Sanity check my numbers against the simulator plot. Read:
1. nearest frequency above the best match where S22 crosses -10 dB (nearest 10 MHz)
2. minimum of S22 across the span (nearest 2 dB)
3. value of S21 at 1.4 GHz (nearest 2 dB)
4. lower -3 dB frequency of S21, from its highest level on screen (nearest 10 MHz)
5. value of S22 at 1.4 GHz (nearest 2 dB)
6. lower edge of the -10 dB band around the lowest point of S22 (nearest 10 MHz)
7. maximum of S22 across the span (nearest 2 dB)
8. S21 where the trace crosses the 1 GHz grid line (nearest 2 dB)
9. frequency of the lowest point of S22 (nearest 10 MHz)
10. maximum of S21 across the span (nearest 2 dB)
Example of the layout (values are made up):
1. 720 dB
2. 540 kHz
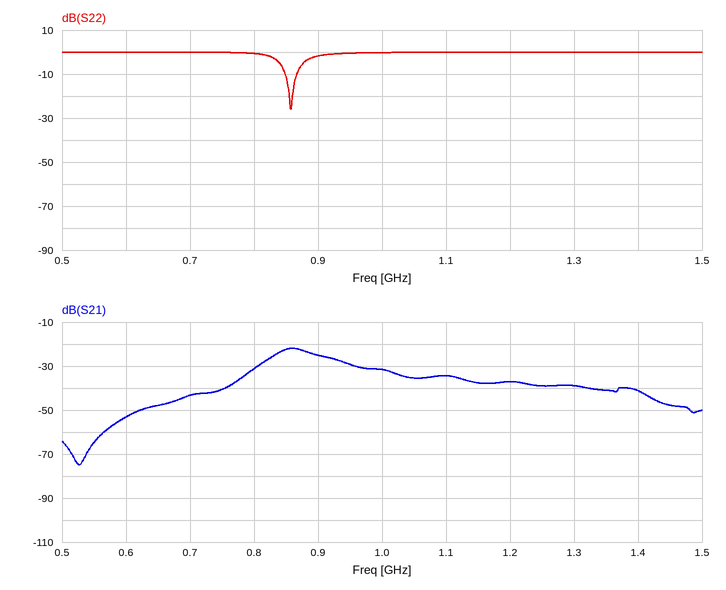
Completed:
1. 870 MHz
2. -26 dB
3. -42 dB
4. 830 MHz
5. 0 dB
6. 850 MHz
7. 0 dB
8. -32 dB
9. 860 MHz
10. -22 dB
